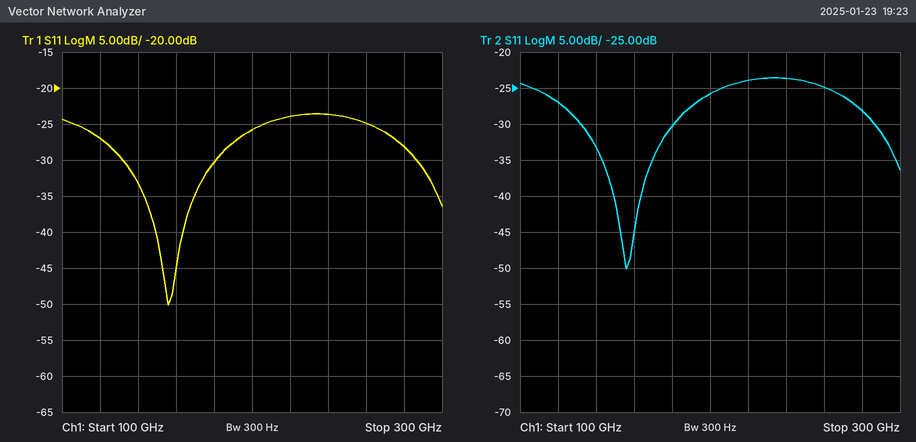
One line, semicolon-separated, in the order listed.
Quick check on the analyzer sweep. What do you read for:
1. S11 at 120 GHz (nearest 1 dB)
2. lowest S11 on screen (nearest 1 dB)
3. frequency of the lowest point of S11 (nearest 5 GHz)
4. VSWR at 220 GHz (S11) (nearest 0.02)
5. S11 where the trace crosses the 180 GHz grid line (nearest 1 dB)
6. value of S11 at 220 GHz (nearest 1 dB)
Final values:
-27 dB; -50 dB; 155 GHz; 1.14; -30 dB; -24 dB
